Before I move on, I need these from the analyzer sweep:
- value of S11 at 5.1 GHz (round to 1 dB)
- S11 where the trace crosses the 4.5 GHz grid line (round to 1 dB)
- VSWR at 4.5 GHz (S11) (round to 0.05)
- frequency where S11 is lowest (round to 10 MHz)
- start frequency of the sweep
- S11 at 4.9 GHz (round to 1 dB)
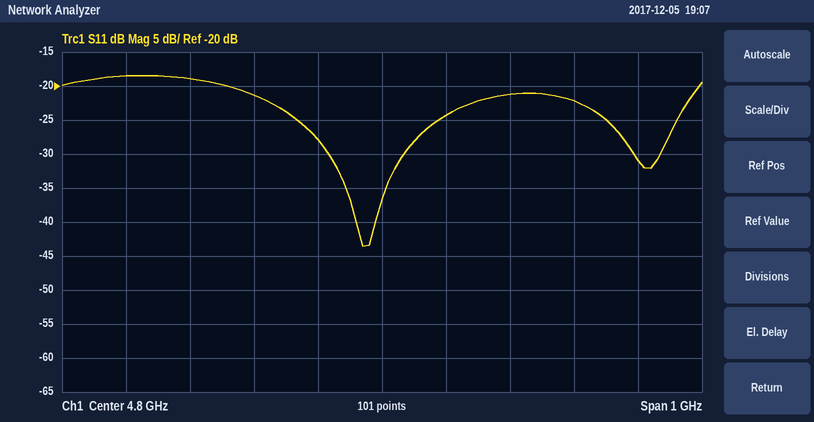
-22 dB
-19 dB
1.25
4.77 GHz
4.3 GHz
-24 dB
